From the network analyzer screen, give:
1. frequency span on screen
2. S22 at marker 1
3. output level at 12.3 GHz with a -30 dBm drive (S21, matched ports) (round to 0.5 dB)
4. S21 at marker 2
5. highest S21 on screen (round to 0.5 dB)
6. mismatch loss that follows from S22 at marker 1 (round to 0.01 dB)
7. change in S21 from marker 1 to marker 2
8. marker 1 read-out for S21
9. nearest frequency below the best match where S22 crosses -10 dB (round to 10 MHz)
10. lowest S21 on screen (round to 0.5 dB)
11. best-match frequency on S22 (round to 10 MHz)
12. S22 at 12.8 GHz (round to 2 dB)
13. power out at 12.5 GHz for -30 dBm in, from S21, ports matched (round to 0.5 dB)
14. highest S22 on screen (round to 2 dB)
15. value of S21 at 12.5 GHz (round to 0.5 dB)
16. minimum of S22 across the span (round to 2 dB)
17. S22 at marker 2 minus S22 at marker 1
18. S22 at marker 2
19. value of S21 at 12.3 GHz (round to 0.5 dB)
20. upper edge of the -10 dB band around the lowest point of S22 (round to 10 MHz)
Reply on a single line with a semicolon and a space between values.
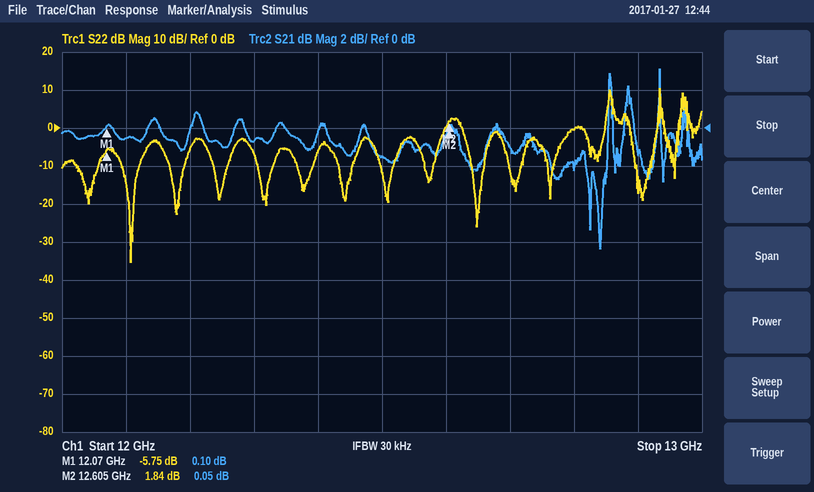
1 GHz; -5.75 dB; -30.5 dBm; 0.05 dB; 3.0 dB; 1.34 dB; -0.05 dB; 0.10 dB; 12.09 GHz; -6.5 dB; 12.11 GHz; 0 dB; -31.5 dBm; 10 dB; -1.5 dB; -36 dB; 7.59 dB; 1.84 dB; -0.5 dB; 12.12 GHz
